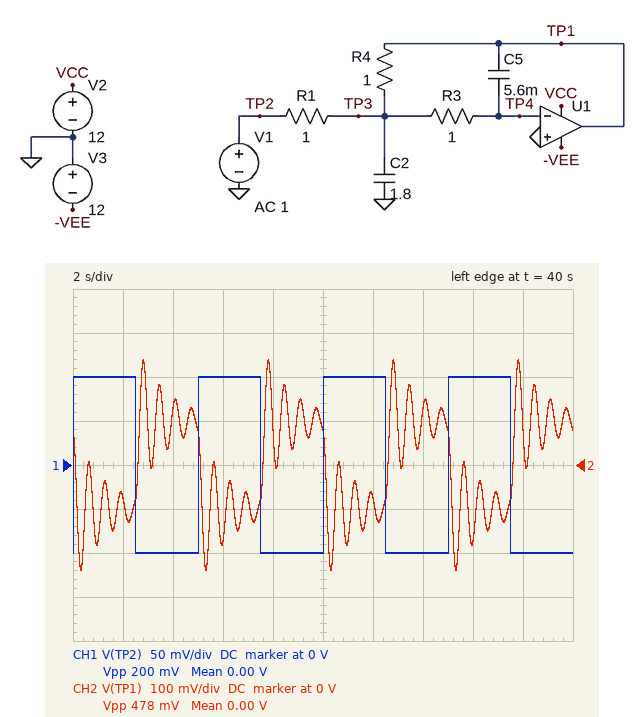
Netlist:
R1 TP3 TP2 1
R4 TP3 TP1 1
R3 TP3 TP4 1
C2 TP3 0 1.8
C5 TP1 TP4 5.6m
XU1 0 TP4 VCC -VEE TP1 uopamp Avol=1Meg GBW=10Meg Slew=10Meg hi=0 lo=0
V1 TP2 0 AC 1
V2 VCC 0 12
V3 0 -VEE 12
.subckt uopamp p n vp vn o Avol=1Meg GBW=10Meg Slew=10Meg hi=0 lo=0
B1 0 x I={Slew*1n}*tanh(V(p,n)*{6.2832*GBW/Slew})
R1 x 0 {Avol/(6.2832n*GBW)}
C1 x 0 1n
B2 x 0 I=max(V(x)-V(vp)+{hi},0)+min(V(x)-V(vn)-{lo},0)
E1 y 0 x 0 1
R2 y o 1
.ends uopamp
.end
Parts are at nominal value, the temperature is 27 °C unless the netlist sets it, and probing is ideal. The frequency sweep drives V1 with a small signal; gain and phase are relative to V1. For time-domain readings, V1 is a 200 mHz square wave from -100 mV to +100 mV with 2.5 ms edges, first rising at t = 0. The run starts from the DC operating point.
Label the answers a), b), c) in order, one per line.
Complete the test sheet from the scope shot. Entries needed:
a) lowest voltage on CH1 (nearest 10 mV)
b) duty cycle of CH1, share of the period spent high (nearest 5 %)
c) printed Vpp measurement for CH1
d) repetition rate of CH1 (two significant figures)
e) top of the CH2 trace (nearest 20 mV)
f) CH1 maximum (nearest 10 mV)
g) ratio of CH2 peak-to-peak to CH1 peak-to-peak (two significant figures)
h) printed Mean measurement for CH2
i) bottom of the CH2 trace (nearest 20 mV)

a) -100 mV
b) 50 %
c) 200 mV
d) 200 mHz
e) 240 mV
f) 100 mV
g) 2.4
h) 0.00 V
i) -240 mV
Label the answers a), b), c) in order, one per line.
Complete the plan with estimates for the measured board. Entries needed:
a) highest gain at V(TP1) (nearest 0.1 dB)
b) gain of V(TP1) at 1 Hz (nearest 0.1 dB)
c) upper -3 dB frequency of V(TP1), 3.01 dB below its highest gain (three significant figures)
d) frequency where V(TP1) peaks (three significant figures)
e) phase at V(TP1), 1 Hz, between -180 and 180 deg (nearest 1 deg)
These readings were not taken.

a) 15.6 dB
b) 4.3 dB
c) 1.70 Hz
d) 1.57 Hz
e) 170 deg
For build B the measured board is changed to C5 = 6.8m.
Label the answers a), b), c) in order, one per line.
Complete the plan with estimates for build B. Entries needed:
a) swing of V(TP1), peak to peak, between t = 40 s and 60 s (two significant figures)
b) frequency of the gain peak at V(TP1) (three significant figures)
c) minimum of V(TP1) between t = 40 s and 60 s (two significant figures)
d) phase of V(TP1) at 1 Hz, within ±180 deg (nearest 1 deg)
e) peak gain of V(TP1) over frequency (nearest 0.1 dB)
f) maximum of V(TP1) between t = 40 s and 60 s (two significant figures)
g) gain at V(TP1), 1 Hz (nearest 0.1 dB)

a) 540 mV
b) 1.43 Hz
c) -270 mV
d) 166 deg
e) 14.7 dB
f) 270 mV
g) 5.5 dB
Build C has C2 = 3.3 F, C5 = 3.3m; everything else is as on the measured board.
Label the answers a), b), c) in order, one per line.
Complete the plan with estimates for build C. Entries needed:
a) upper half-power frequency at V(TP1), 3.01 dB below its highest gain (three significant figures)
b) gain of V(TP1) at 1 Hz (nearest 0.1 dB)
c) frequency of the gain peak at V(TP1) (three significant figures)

a) 1.59 Hz
b) 4.8 dB
c) 1.52 Hz
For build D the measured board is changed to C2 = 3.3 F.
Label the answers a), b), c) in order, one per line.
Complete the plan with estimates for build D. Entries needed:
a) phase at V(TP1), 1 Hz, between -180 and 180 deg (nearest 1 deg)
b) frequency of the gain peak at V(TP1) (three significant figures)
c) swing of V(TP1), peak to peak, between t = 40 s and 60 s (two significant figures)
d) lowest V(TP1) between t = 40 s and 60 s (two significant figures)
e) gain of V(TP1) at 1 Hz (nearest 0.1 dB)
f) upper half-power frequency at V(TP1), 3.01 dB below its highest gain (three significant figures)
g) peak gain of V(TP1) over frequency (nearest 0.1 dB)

a) 159 deg
b) 1.17 Hz
c) 460 mV
d) -230 mV
e) 10.7 dB
f) 1.24 Hz
g) 18.2 dB
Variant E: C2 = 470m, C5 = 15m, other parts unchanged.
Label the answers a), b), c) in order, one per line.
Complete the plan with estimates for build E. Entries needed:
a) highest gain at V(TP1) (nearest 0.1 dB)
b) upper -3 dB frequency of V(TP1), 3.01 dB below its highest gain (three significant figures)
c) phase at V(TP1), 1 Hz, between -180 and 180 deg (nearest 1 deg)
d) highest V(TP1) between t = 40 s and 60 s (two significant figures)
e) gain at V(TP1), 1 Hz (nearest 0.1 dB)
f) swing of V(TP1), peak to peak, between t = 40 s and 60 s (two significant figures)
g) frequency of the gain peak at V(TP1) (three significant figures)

a) 5.7 dB
b) 2.22 Hz
c) 159 deg
d) 180 mV
e) 2.2 dB
f) 370 mV
g) 1.75 Hz
